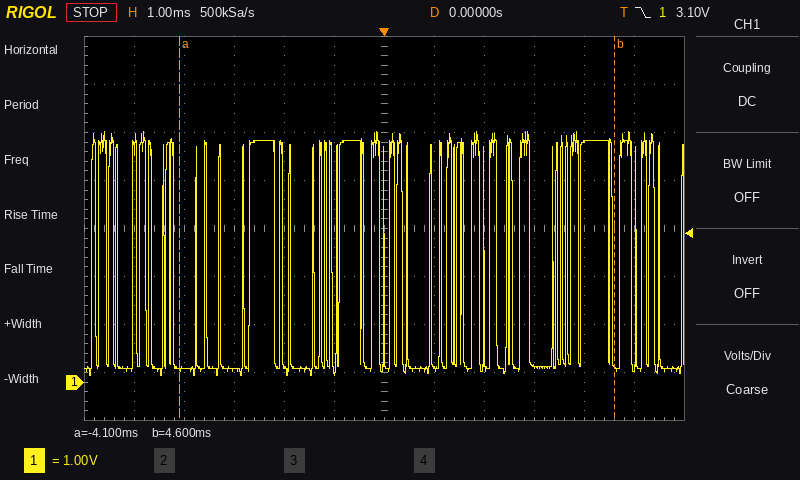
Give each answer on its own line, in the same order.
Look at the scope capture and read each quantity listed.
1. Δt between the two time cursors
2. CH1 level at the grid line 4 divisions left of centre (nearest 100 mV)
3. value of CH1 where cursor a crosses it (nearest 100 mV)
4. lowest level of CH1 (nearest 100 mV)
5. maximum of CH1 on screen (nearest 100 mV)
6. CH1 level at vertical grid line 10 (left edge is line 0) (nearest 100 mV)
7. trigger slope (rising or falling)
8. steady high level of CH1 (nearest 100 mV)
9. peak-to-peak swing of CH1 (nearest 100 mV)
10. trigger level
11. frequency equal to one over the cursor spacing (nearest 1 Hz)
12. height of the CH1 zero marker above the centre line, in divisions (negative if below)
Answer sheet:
8.7 ms
300 mV
300 mV
100 mV
5.2 V
5.0 V
falling
5.0 V
5.1 V
3.10 V
115 Hz
-3.2 div
